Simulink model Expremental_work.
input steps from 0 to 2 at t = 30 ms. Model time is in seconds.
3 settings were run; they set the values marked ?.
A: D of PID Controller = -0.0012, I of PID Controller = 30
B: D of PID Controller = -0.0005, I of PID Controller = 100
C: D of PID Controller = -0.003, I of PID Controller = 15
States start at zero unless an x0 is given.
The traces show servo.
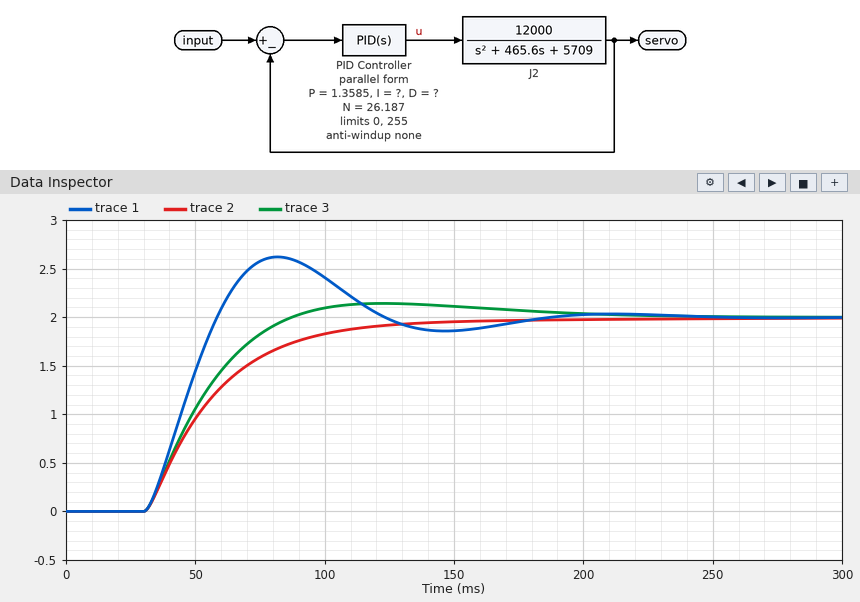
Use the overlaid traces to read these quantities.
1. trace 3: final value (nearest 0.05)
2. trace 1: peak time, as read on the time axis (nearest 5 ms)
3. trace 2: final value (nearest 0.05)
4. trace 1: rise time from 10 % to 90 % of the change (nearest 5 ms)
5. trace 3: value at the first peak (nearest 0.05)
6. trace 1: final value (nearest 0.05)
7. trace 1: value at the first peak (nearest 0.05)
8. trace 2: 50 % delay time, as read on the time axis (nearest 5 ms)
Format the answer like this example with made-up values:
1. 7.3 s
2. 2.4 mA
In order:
1. 2.00
2. 80 ms
3. 2.00
4. 20 ms
5. 2.15
6. 2.00
7. 2.60
8. 50 ms
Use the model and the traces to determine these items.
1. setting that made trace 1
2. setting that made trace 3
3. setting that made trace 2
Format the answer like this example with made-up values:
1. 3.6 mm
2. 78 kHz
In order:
1. B
2. A
3. C
